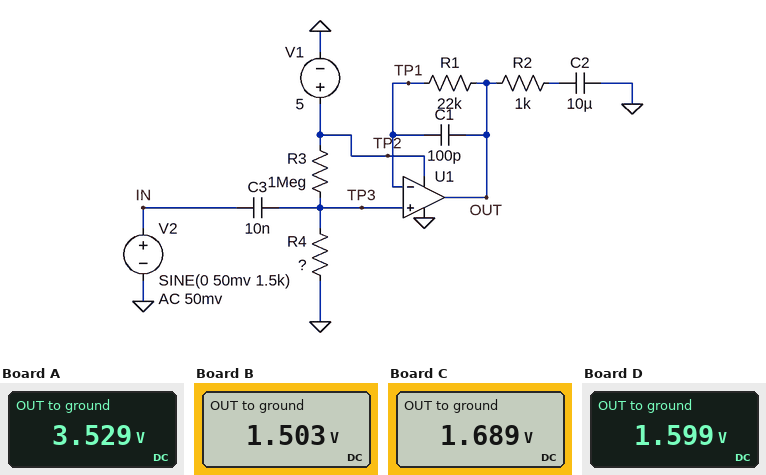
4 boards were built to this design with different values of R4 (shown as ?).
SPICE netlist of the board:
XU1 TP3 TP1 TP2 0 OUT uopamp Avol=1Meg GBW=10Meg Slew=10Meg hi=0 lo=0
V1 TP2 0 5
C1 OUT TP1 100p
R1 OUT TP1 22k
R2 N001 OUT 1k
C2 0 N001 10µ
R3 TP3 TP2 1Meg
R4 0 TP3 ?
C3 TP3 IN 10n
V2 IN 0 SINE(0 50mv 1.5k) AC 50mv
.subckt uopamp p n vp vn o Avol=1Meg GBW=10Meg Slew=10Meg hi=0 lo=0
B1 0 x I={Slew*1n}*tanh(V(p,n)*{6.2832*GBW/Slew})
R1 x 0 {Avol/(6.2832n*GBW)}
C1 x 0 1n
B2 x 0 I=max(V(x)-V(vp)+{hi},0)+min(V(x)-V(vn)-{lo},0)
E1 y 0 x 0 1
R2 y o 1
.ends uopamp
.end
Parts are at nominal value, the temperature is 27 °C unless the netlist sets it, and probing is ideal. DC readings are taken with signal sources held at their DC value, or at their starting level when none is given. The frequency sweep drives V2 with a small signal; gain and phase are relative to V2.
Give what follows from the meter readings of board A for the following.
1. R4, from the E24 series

2.4 MΩ
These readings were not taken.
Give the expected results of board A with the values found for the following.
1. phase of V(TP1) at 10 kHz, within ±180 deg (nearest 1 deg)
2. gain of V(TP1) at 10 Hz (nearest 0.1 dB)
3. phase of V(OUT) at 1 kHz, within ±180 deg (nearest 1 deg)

0 deg
-7.8 dB
1 deg
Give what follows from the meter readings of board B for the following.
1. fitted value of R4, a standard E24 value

430 kΩ
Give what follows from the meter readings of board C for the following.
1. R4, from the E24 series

510 kΩ
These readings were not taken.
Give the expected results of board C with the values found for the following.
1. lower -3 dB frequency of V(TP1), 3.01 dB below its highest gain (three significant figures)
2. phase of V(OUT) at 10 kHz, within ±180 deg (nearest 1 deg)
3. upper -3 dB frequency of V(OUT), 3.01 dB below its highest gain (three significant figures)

47.1 Hz
0 deg
9.99 MHz
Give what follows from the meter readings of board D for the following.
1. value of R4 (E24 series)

470 kΩ
